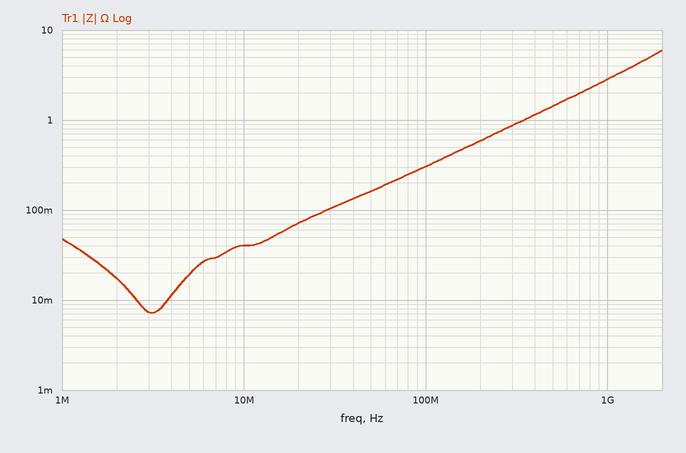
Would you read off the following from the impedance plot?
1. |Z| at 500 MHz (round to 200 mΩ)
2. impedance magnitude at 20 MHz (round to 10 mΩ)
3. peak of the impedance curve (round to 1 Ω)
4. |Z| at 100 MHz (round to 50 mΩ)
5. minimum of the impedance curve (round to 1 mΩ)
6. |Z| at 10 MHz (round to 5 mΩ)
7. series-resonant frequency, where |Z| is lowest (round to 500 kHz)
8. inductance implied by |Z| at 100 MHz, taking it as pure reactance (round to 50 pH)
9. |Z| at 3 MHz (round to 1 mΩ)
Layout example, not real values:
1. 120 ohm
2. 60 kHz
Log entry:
1. 1.4 Ω
2. 70 mΩ
3. 6 Ω
4. 300 mΩ
5. 7 mΩ
6. 40 mΩ
7. 3.0 MHz
8. 500 pH
9. 7 mΩ
